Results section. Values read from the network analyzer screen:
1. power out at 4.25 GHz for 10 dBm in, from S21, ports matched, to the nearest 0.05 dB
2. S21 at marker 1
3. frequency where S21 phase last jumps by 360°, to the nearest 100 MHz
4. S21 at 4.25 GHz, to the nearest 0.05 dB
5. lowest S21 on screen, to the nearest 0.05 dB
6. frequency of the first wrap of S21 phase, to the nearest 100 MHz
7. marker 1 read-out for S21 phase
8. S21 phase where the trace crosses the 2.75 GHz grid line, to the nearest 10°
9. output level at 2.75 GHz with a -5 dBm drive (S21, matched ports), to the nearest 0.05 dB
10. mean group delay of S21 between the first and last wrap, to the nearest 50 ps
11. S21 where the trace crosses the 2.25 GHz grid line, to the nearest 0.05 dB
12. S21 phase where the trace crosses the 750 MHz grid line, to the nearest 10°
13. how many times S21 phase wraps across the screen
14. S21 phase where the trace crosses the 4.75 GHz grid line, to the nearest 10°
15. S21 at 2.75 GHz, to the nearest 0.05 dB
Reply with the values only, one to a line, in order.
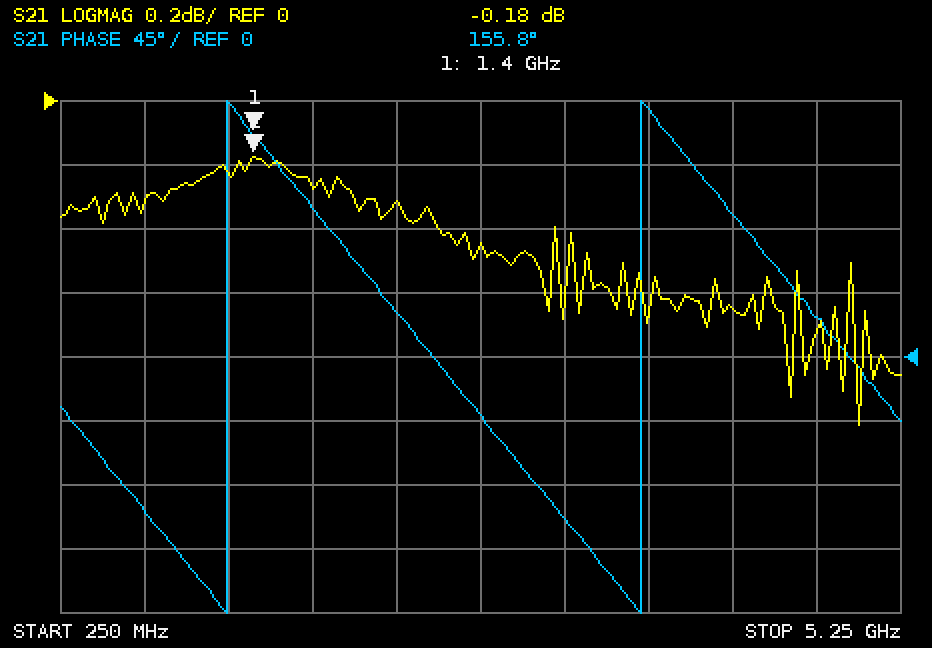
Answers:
9.35 dBm
-0.18 dB
3.7 GHz
-0.65 dB
-1.00 dB
1.2 GHz
155.8°
-40°
-5.45 dBm
400 ps
-0.30 dB
-110°
2
30°
-0.45 dB
